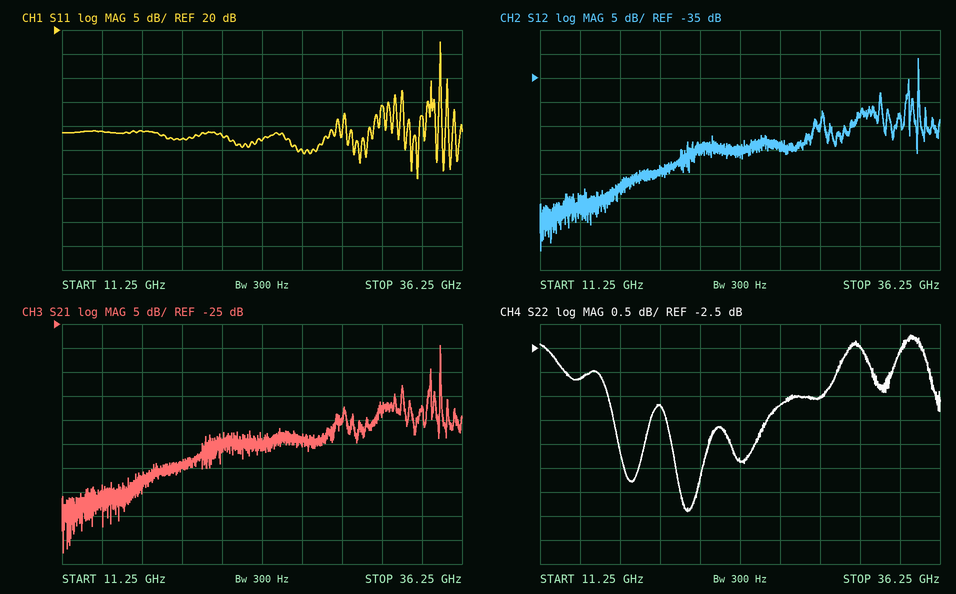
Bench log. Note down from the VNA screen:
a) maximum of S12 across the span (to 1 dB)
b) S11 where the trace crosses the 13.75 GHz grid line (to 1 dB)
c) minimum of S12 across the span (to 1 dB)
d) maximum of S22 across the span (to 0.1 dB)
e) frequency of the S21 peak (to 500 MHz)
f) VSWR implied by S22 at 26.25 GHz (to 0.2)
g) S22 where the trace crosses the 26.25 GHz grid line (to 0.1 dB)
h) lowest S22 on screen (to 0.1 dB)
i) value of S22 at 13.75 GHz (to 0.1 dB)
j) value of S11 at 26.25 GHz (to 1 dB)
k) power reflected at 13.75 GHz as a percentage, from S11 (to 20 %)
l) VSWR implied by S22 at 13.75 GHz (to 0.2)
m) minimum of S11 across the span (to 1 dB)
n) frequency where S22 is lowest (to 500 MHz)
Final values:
-31 dB
-1 dB
-71 dB
-2.2 dB
35.0 GHz
4.8
-3.7 dB
-5.9 dB
-3.1 dB
-5 dB
80 %
5.6
-11 dB
20.5 GHz
